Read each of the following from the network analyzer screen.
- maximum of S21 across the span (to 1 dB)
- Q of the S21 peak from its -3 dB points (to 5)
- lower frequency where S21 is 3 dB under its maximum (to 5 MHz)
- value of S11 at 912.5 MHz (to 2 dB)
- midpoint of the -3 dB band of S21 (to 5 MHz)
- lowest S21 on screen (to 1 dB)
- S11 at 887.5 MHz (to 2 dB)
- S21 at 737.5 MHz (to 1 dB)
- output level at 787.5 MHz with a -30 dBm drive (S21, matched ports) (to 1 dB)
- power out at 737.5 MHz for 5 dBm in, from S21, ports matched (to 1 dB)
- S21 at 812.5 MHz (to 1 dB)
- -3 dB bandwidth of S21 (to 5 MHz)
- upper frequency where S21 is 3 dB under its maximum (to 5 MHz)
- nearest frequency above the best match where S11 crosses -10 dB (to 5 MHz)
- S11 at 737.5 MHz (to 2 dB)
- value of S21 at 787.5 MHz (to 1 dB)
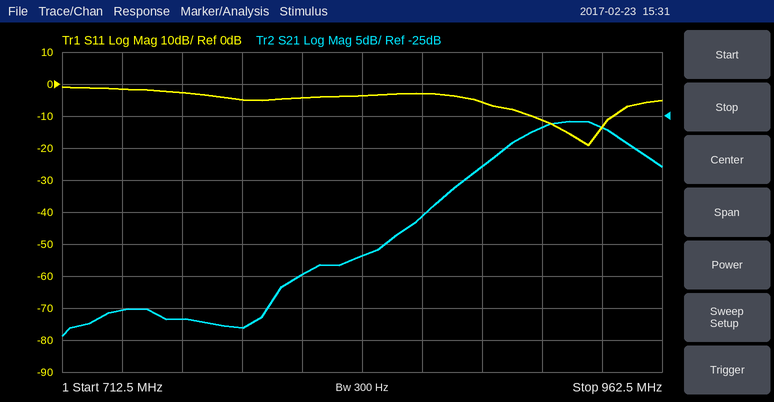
-26 dB
20
900 MHz
-12 dB
925 MHz
-59 dB
-6 dB
-55 dB
-88 dBm
-50 dBm
-50 dB
45 MHz
945 MHz
940 MHz
-2 dB
-58 dB
